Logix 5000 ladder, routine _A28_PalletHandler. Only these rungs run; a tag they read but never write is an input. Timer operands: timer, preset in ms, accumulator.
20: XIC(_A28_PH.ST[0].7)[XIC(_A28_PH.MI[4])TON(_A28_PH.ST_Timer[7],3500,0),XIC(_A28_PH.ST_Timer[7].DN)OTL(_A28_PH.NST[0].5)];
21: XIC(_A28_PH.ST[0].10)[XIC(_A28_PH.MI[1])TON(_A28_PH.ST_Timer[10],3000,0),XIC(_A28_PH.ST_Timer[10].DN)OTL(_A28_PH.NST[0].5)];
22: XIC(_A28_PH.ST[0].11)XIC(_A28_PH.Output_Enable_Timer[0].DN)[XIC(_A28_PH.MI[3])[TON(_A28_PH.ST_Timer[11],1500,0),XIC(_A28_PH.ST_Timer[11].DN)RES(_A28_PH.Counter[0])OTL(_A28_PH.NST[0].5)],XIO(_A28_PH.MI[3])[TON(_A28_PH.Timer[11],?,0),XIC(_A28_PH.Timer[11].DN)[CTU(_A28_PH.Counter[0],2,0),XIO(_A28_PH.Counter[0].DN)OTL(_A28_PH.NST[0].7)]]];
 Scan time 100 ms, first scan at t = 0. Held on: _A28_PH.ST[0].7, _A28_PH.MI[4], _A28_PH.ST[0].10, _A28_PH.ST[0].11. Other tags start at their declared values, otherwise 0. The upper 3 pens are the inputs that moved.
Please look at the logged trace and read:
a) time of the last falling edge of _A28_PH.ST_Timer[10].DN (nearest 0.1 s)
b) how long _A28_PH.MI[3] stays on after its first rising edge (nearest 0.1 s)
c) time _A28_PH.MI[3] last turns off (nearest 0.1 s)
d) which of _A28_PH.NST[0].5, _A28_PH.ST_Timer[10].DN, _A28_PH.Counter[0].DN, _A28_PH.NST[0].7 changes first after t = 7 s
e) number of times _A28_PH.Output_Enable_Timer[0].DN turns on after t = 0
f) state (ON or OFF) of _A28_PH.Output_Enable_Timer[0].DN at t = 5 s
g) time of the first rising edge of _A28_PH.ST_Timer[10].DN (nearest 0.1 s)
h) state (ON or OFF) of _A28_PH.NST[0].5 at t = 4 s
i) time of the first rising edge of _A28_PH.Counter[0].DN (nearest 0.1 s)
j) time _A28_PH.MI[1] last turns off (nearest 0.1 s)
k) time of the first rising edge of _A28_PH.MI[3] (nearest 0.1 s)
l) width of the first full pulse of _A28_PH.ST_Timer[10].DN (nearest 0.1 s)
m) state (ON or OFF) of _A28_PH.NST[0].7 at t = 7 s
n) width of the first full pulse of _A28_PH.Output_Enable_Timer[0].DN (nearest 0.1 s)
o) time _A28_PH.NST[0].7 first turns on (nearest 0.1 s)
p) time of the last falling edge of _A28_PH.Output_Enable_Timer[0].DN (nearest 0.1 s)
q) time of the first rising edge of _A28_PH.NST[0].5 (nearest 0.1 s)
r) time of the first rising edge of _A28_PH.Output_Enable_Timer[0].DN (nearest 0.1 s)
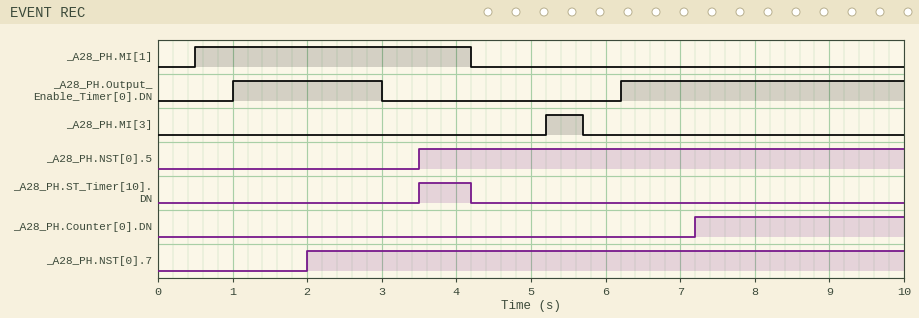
4.2 s
0.5 s
5.7 s
_A28_PH.Counter[0].DN
2
OFF
3.5 s
ON
7.2 s
4.2 s
5.2 s
0.7 s
ON
2.0 s
2.0 s
3.0 s
3.5 s
1.0 s
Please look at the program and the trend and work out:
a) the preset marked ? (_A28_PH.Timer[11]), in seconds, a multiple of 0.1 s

1.0 s
